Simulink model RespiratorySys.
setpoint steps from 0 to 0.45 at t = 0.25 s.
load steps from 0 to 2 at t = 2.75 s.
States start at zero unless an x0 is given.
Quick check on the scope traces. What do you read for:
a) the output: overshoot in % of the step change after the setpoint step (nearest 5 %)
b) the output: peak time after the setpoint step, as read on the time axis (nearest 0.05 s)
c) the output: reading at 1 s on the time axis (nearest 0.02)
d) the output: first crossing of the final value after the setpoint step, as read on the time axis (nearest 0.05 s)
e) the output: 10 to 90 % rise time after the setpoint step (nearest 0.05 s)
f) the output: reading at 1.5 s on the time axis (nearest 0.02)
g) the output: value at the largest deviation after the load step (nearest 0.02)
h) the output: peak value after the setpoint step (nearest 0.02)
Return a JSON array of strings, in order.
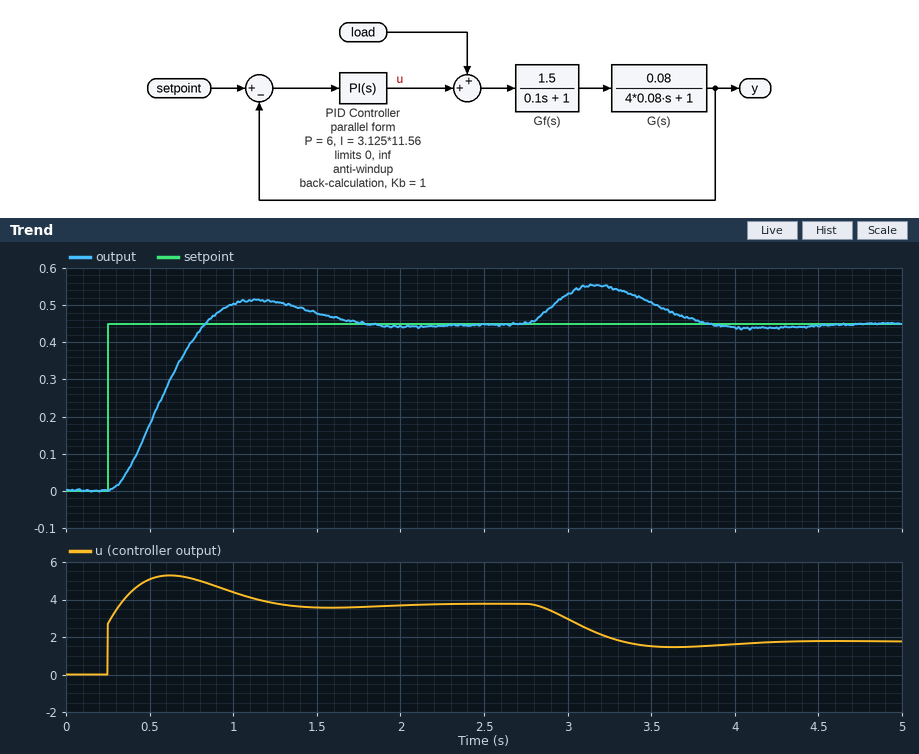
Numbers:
["15 %", "1.15 s", "0.50", "0.85 s", "0.40 s", "0.48", "0.56", "0.52"]
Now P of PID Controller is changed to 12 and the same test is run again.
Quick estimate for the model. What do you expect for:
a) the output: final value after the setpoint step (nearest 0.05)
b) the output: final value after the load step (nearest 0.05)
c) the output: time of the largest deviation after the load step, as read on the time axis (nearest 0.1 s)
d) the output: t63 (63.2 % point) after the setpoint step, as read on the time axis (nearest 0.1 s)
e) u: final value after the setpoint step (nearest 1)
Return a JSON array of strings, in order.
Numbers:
["0.45", "0.45", "3.1 s", "0.5 s", "4"]
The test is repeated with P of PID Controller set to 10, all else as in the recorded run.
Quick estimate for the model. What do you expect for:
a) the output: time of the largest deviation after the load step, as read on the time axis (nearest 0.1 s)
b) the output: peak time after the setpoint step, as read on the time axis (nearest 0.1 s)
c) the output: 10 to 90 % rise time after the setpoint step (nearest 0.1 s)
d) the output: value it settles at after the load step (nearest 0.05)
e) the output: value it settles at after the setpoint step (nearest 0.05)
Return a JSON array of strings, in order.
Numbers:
["3.1 s", "1.0 s", "0.4 s", "0.45", "0.45"]
